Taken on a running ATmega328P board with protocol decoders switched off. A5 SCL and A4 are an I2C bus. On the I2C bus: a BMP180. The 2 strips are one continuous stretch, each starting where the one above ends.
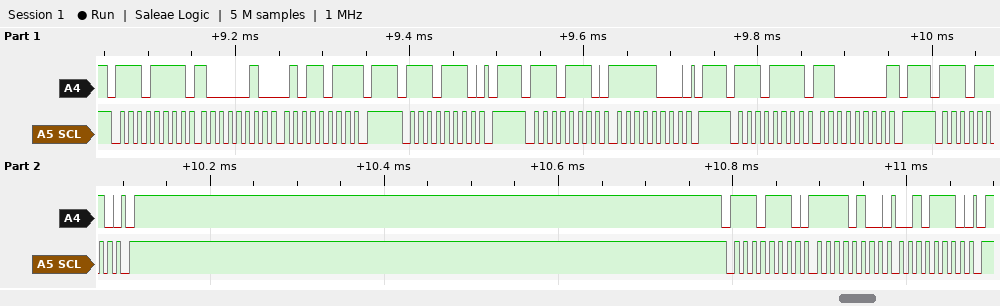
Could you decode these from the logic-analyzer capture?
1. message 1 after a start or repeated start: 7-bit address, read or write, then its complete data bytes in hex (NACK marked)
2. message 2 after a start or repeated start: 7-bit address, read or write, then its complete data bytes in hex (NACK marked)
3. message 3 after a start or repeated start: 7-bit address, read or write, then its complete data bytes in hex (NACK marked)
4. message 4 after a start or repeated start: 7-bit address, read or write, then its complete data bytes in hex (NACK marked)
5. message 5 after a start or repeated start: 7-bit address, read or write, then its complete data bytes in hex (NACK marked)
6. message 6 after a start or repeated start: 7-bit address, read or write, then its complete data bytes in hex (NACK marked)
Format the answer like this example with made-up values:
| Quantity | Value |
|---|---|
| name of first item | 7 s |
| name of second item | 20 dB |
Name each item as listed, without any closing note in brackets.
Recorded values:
| Quantity | Value |
|---|---|
| message 1 after a start or repeated start: 7-bit address, read or write, then its complete data bytes in hex | 0x77 read: 82 5B NACK |
| message 2 after a start or repeated start: 7-bit address, read or write, then its complete data bytes in hex | 0x77 write |
| message 3 after a start or repeated start: 7-bit address, read or write, then its complete data bytes in hex | 0x77 write: F8 |
| message 4 after a start or repeated start: 7-bit address, read or write, then its complete data bytes in hex | 0x77 read: C0 NACK |
| message 5 after a start or repeated start: 7-bit address, read or write, then its complete data bytes in hex | 0x77 write |
| message 6 after a start or repeated start: 7-bit address, read or write, then its complete data bytes in hex | 0x77 write: F4 2E |
